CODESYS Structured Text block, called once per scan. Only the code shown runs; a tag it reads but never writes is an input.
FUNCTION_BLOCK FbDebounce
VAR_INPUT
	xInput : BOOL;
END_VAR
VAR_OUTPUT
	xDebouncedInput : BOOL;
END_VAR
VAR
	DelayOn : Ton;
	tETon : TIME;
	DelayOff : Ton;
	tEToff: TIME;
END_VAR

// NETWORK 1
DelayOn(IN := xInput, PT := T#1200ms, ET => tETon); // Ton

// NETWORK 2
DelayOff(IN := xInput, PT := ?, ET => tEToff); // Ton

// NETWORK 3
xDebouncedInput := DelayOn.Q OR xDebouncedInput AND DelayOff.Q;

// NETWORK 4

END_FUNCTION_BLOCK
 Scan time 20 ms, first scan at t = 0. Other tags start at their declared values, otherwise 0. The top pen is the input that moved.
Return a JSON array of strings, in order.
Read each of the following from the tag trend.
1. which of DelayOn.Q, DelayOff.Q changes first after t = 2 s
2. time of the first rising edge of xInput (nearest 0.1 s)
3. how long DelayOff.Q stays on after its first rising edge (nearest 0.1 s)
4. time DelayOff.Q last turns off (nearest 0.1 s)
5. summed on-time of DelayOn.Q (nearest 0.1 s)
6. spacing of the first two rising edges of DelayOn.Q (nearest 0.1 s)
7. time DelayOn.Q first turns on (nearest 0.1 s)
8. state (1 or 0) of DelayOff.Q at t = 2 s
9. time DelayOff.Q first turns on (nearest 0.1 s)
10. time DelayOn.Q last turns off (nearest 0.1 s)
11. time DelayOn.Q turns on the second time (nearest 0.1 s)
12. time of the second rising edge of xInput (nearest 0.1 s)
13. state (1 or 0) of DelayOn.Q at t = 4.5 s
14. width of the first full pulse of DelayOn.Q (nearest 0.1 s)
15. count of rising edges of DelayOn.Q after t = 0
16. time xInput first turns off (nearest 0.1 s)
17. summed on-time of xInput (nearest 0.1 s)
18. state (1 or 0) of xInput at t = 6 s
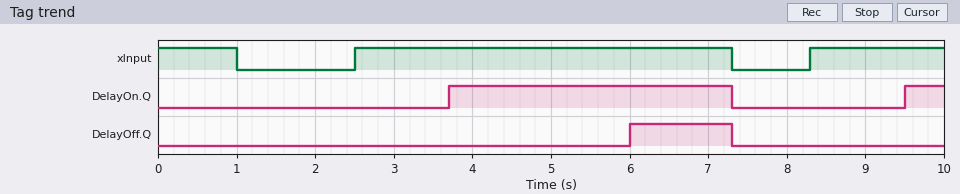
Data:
["DelayOn.Q", "2.5 s", "1.3 s", "7.3 s", "4.1 s", "5.8 s", "3.7 s", "0", "6.0 s", "7.3 s", "9.5 s", "8.3 s", "1", "3.6 s", "2", "1.0 s", "7.5 s", "1"]
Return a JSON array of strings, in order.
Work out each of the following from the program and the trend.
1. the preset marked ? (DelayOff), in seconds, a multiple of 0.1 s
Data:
["3.5 s"]
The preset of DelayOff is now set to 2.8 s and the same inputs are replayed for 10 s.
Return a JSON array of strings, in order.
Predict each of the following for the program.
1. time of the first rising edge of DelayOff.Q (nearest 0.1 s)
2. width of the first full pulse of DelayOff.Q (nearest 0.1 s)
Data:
["5.3 s", "2.0 s"]
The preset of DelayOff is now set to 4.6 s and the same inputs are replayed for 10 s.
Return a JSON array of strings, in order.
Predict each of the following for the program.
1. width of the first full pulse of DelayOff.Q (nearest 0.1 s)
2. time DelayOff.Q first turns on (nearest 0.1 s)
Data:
["0.2 s", "7.1 s"]
